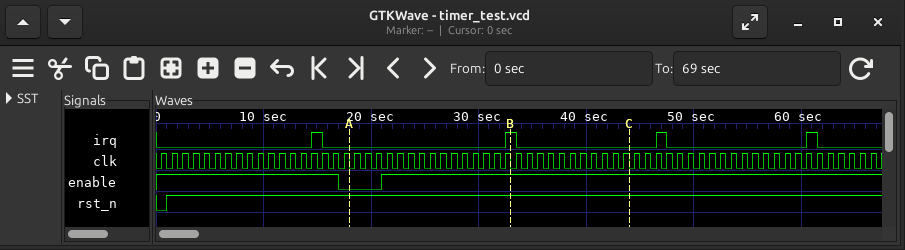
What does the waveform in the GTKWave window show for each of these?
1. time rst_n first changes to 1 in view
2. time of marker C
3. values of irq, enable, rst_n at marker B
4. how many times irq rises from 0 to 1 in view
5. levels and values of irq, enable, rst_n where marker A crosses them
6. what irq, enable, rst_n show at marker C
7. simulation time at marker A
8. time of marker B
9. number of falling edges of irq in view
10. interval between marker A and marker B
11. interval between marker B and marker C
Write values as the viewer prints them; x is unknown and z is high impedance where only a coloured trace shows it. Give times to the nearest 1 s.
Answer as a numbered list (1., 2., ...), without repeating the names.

1. 1 s
2. 44 s
3. irq=1, enable=1, rst_n=1
4. 4
5. irq=0, enable=0, rst_n=1
6. irq=0, enable=1, rst_n=1
7. 18 s
8. 33 s
9. 4
10. 15 s
11. 11 s
